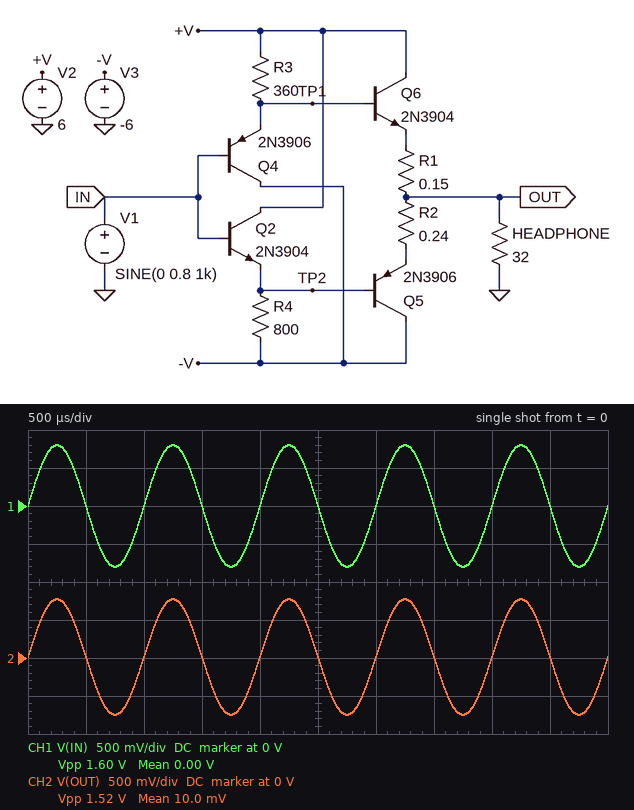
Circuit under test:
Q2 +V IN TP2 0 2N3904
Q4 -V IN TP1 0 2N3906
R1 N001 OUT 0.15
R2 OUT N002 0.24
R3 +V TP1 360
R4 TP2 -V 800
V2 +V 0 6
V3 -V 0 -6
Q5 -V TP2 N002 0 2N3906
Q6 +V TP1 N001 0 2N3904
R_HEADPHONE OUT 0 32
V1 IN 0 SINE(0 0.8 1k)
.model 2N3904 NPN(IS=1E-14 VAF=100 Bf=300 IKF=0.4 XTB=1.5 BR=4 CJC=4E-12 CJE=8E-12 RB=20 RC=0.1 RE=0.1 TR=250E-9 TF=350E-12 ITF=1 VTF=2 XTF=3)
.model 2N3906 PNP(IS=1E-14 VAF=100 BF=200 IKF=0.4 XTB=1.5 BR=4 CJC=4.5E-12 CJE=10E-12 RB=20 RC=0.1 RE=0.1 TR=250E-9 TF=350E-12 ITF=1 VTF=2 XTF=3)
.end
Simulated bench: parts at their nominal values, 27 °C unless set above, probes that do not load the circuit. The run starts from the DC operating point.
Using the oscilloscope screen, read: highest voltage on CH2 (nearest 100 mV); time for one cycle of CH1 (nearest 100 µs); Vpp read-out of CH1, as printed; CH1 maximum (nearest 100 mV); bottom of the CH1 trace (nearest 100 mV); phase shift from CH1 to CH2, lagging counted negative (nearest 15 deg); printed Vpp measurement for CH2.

800 mV
1.0 ms
1.60 V
800 mV
-800 mV
0 deg
1.52 V
